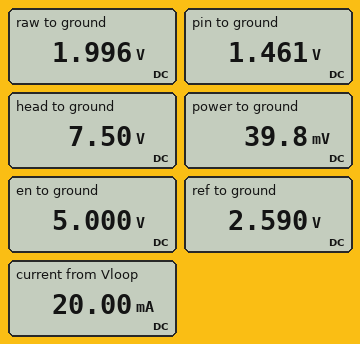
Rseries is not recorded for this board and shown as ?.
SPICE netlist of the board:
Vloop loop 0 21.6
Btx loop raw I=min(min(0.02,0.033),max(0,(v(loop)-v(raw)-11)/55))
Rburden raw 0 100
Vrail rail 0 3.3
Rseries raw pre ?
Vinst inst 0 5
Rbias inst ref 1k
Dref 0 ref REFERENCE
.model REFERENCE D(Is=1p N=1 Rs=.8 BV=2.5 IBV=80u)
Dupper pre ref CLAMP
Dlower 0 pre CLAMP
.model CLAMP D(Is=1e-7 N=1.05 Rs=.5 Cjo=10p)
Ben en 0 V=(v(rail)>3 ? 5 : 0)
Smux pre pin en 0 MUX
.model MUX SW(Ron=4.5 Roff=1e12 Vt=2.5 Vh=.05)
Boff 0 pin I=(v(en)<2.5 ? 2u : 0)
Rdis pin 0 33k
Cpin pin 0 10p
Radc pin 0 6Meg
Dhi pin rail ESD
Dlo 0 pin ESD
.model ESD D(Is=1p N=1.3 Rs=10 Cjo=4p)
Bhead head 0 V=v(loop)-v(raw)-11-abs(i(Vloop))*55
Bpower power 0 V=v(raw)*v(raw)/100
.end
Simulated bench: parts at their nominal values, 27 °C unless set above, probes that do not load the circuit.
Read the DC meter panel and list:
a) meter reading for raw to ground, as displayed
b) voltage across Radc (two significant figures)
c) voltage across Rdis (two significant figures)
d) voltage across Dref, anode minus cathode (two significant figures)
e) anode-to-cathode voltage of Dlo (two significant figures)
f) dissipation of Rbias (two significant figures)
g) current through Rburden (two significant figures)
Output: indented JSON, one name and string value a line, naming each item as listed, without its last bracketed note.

{
  "meter reading for raw to ground, as displayed": "1.996 V",
  "voltage across Radc": "1.5 V",
  "voltage across Rdis": "1.5 V",
  "voltage across Dref, anode minus cathode": "-2.6 V",
  "anode-to-cathode voltage of Dlo": "-1.5 V",
  "dissipation of Rbias": "5.8 mW",
  "current through Rburden": "20 mA"
}
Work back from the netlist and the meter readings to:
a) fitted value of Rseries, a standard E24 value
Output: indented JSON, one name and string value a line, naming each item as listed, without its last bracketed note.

{
  "fitted value of Rseries, a standard E24 value": "12 kΩ"
}
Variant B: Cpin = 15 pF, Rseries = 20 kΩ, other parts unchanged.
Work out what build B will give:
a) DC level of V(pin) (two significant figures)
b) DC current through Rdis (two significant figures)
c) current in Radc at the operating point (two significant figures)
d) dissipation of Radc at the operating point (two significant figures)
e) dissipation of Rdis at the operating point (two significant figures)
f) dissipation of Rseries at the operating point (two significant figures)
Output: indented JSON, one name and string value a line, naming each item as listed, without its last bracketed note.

{
  "DC level of V(pin)": "1.2 V",
  "DC current through Rdis": "38 µA",
  "current in Radc at the operating point": "210 nA",
  "dissipation of Radc at the operating point": "260 nW",
  "dissipation of Rdis at the operating point": "47 µW",
  "dissipation of Rseries at the operating point": "29 µW"
}
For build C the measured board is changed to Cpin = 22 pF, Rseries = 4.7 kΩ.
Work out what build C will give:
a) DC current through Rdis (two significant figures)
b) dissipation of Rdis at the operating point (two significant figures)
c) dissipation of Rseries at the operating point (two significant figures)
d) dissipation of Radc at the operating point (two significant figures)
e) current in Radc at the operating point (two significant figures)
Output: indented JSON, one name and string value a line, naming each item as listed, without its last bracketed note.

{
  "DC current through Rdis": "53 µA",
  "dissipation of Rdis at the operating point": "92 µW",
  "dissipation of Rseries at the operating point": "13 µW",
  "dissipation of Radc at the operating point": "510 nW",
  "current in Radc at the operating point": "290 nA"
}
